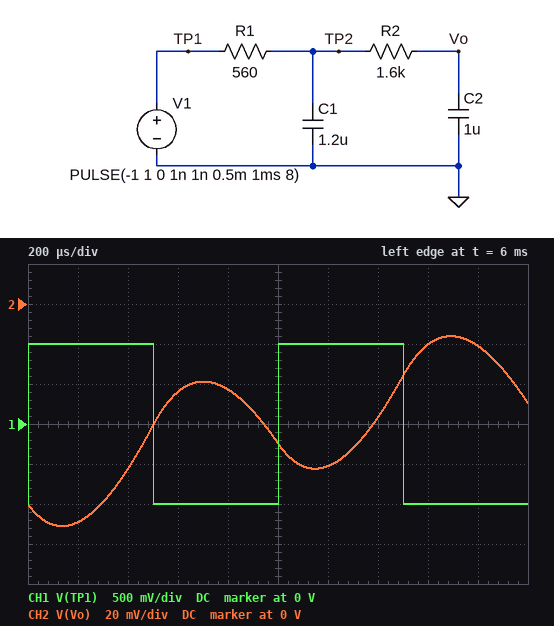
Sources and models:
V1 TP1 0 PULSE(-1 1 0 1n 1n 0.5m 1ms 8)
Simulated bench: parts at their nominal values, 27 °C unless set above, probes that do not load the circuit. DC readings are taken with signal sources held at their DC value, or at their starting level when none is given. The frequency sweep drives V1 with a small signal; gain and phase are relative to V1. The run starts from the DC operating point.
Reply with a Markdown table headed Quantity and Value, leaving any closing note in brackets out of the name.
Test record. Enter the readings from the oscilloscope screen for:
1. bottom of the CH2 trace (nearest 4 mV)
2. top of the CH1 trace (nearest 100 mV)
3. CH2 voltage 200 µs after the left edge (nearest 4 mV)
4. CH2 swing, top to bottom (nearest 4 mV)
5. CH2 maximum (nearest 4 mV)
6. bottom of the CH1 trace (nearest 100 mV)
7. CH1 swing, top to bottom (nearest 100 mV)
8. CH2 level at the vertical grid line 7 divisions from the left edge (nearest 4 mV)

| Quantity | Value |
|---|---|
| bottom of the CH2 trace | -112 mV |
| top of the CH1 trace | 1.0 V |
| CH2 voltage 200 µs after the left edge | -108 mV |
| CH2 swing, top to bottom | 96 mV |
| CH2 maximum | -16 mV |
| bottom of the CH1 trace | -1.0 V |
| CH1 swing, top to bottom | 2.0 V |
| CH2 level at the vertical grid line 7 divisions from the left edge | -56 mV |
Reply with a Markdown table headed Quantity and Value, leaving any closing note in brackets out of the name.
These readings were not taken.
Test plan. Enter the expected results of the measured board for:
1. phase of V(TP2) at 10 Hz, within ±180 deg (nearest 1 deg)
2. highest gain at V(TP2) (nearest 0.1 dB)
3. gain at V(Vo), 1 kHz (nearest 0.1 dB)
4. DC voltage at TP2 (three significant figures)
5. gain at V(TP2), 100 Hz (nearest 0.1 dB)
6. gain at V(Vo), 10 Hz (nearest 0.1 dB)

| Quantity | Value |
|---|---|
| phase of V(TP2) at 10 Hz, within ±180 deg | -4 deg |
| highest gain at V(TP2) | 0 dB |
| gain at V(Vo), 1 kHz | -33.1 dB |
| DC voltage at TP2 | -1.00 V |
| gain at V(TP2), 100 Hz | -2.4 dB |
| gain at V(Vo), 10 Hz | -0.1 dB |
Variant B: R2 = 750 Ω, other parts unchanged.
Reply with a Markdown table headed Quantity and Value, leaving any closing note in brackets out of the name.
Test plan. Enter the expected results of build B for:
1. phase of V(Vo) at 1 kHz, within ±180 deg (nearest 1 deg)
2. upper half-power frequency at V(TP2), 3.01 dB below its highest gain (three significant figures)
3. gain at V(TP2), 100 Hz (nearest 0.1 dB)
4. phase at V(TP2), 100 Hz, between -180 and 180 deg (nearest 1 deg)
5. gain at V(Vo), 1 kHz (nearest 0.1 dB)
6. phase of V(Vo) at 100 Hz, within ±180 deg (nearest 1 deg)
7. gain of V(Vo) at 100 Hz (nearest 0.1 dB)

| Quantity | Value |
|---|---|
| phase of V(Vo) at 1 kHz, within ±180 deg | -147 deg |
| upper half-power frequency at V(TP2), 3.01 dB below its highest gain | 115 Hz |
| gain at V(TP2), 100 Hz | -2.5 dB |
| phase at V(TP2), 100 Hz, between -180 and 180 deg | -32 deg |
| gain at V(Vo), 1 kHz | -27.1 dB |
| phase of V(Vo) at 100 Hz, within ±180 deg | -57 deg |
| gain of V(Vo) at 100 Hz | -3.4 dB |
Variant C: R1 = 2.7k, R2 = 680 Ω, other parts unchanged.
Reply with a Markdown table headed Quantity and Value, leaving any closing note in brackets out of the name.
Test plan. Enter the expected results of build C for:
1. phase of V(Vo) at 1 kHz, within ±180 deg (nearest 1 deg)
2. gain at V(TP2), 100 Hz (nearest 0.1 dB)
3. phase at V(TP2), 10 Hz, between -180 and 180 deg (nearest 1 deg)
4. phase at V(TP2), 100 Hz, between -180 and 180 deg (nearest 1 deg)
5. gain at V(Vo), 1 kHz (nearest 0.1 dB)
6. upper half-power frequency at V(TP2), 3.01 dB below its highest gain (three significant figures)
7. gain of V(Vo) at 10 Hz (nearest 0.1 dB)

| Quantity | Value |
|---|---|
| phase of V(Vo) at 1 kHz, within ±180 deg | -154 deg |
| gain at V(TP2), 100 Hz | -11.7 dB |
| phase at V(TP2), 10 Hz, between -180 and 180 deg | -20 deg |
| phase at V(TP2), 100 Hz, between -180 and 180 deg | -65 deg |
| gain at V(Vo), 1 kHz | -39.6 dB |
| upper half-power frequency at V(TP2), 3.01 dB below its highest gain | 25.6 Hz |
| gain of V(Vo) at 10 Hz | -0.6 dB |
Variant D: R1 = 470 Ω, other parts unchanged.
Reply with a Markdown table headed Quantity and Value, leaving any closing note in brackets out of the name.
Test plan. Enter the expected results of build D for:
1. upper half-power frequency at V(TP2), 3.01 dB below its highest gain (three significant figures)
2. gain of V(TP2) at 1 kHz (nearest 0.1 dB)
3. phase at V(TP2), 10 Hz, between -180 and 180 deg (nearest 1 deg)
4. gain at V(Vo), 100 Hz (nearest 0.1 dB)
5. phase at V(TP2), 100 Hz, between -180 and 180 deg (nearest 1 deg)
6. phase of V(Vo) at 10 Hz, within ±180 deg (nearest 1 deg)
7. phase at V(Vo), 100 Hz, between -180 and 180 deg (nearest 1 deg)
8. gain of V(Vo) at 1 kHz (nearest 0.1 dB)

| Quantity | Value |
|---|---|
| upper half-power frequency at V(TP2), 3.01 dB below its highest gain | 167 Hz |
| gain of V(TP2) at 1 kHz | -11.6 dB |
| phase at V(TP2), 10 Hz, between -180 and 180 deg | -4 deg |
| gain at V(Vo), 100 Hz | -5.0 dB |
| phase at V(TP2), 100 Hz, between -180 and 180 deg | -24 deg |
| phase of V(Vo) at 10 Hz, within ±180 deg | -9 deg |
| phase at V(Vo), 100 Hz, between -180 and 180 deg | -69 deg |
| gain of V(Vo) at 1 kHz | -31.7 dB |
